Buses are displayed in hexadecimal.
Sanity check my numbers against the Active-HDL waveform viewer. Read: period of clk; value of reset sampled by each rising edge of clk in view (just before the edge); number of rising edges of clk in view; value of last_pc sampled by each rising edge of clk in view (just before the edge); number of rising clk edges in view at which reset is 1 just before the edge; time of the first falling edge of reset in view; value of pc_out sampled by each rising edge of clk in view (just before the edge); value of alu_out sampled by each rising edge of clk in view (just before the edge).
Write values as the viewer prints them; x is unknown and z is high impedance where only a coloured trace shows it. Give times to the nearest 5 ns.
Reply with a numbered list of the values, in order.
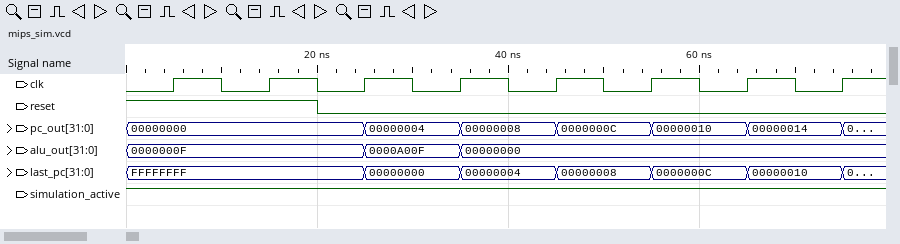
1. 10 ns
2. 1 1 0 0 0 0 0 0
3. 8
4. FFFFFFFF, FFFFFFFF, FFFFFFFF, 00000000, 00000004, 00000008, 0000000C, 00000010
5. 2
6. 20 ns
7. 00000000, 00000000, 00000000, 00000004, 00000008, 0000000C, 00000010, 00000014
8. 0000000F, 0000000F, 0000000F, 0000A00F, 00000000, 00000000, 00000000, 00000000
